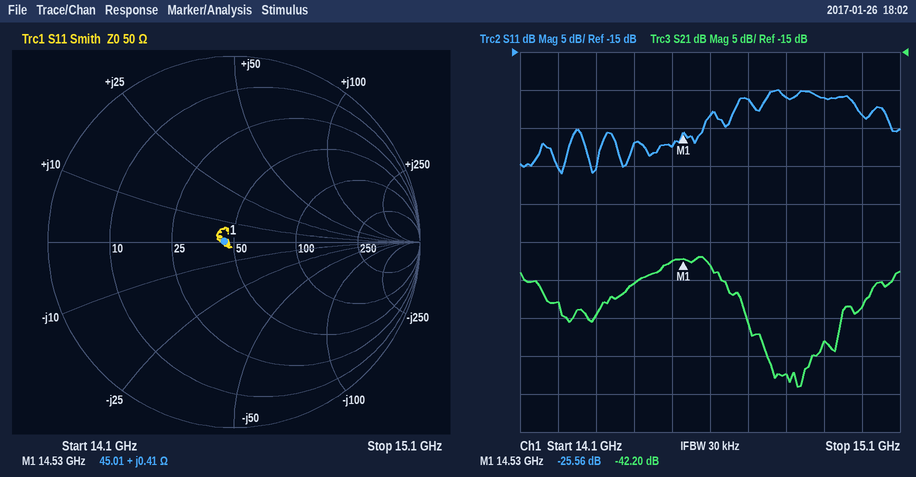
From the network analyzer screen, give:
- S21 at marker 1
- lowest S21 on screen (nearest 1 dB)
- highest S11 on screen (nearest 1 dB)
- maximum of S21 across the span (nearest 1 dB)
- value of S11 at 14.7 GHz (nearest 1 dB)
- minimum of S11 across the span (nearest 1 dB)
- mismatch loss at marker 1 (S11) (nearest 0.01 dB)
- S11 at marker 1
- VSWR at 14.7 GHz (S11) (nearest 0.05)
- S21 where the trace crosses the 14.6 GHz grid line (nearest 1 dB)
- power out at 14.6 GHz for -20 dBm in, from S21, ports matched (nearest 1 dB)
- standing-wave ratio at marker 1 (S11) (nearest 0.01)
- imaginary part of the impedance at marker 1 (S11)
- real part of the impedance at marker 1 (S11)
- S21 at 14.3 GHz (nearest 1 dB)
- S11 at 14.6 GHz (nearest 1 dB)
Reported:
-42.20 dB
-59 dB
-20 dB
-42 dB
-21 dB
-31 dB
0.01 dB
-25.56 dB
1.20
-43 dB
-63 dBm
1.11
+0.41 Ω
45.01 Ω
-50 dB
-23 dB
